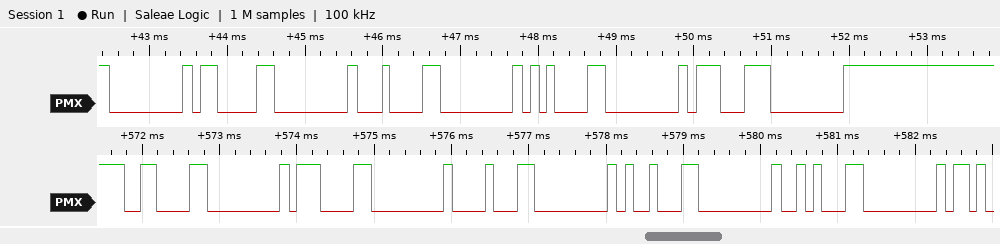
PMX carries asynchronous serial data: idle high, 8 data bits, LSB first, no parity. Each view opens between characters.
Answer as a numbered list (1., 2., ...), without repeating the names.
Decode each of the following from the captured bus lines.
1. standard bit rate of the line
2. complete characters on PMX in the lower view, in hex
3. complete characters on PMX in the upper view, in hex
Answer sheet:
1. 9600 baud
2. 86, 00, 87, 00, 88, 00, 89, 00, 8A, 00
3. 00, 83, 00, 84, 00, 85, 00, C7, 00
